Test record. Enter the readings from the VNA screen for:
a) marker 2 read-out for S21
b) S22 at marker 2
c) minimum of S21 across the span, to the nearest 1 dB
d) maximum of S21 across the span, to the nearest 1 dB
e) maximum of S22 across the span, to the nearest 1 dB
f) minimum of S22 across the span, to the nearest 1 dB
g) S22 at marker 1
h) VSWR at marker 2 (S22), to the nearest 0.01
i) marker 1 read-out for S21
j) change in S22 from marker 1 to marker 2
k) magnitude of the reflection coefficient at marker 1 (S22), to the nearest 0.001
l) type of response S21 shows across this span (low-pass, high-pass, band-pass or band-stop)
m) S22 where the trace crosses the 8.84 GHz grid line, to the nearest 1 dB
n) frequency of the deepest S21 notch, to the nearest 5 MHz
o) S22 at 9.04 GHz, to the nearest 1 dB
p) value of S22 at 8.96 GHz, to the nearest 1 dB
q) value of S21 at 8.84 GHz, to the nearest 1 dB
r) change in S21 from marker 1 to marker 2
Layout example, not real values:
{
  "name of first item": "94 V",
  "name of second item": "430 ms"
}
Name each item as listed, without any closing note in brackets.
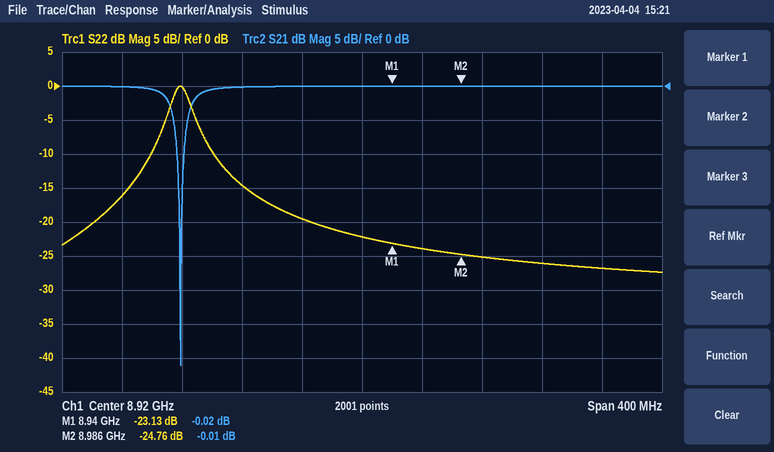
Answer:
{
  "marker 2 read-out for S21": "-0.01 dB",
  "S22 at marker 2": "-24.76 dB",
  "minimum of S21 across the span, to the nearest 1 dB": "-41 dB",
  "maximum of S21 across the span, to the nearest 1 dB": "0 dB",
  "maximum of S22 across the span, to the nearest 1 dB": "0 dB",
  "minimum of S22 across the span, to the nearest 1 dB": "-27 dB",
  "S22 at marker 1": "-23.13 dB",
  "VSWR at marker 2 (S22), to the nearest 0.01": "1.12",
  "marker 1 read-out for S21": "-0.02 dB",
  "change in S22 from marker 1 to marker 2": "-1.63 dB",
  "magnitude of the reflection coefficient at marker 1 (S22), to the nearest 0.001": "0.070",
  "type of response S21 shows across this span": "band-stop",
  "S22 where the trace crosses the 8.84 GHz grid line, to the nearest 1 dB": "-15 dB",
  "frequency of the deepest S21 notch, to the nearest 5 MHz": "8.800 GHz",
  "S22 at 9.04 GHz, to the nearest 1 dB": "-26 dB",
  "value of S22 at 8.96 GHz, to the nearest 1 dB": "-24 dB",
  "value of S21 at 8.84 GHz, to the nearest 1 dB": "0 dB",
  "change in S21 from marker 1 to marker 2": "0.01 dB"
}
